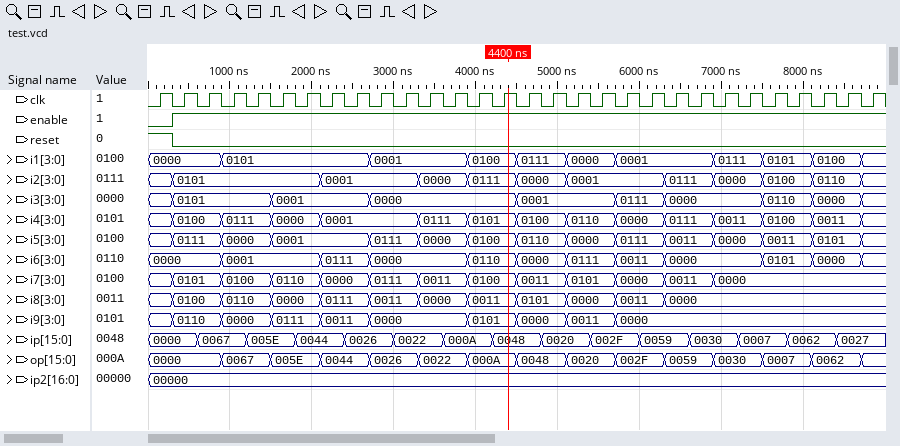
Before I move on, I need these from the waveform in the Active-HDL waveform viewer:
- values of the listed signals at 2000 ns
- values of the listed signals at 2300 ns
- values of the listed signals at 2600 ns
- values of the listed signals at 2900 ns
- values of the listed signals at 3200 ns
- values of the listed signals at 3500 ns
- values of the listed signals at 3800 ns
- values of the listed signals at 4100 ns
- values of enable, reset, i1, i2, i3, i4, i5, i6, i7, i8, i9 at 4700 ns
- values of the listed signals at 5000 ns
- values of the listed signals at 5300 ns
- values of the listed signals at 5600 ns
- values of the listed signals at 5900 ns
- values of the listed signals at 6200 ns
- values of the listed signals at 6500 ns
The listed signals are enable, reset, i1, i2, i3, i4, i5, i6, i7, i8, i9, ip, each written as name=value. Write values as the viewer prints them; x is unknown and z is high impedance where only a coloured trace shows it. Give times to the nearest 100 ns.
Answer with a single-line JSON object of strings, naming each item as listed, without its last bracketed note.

{"values of the listed signals at 2000 ns": "enable=1, reset=0, i1=0101, i2=0101, i3=0001, i4=0000, i5=0001, i6=0001, i7=0110, i8=0000, i9=0111, ip=0044", "values of the listed signals at 2300 ns": "enable=1, reset=0, i1=0101, i2=0001, i3=0001, i4=0001, i5=0001, i6=0111, i7=0000, i8=0111, i9=0011, ip=0044", "values of the listed signals at 2600 ns": "enable=1, reset=0, i1=0101, i2=0001, i3=0001, i4=0001, i5=0001, i6=0111, i7=0000, i8=0111, i9=0011, ip=0026", "values of the listed signals at 2900 ns": "enable=1, reset=0, i1=0001, i2=0001, i3=0000, i4=0001, i5=0111, i6=0000, i7=0111, i8=0011, i9=0000, ip=0026", "values of the listed signals at 3200 ns": "enable=1, reset=0, i1=0001, i2=0001, i3=0000, i4=0001, i5=0111, i6=0000, i7=0111, i8=0011, i9=0000, ip=0022", "values of the listed signals at 3500 ns": "enable=1, reset=0, i1=0001, i2=0000, i3=0000, i4=0111, i5=0000, i6=0000, i7=0011, i8=0000, i9=0000, ip=0022", "values of the listed signals at 3800 ns": "enable=1, reset=0, i1=0001, i2=0000, i3=0000, i4=0111, i5=0000, i6=0000, i7=0011, i8=0000, i9=0000, ip=000A", "values of the listed signals at 4100 ns": "enable=1, reset=0, i1=0100, i2=0111, i3=0000, i4=0101, i5=0100, i6=0110, i7=0100, i8=0011, i9=0101, ip=000A", "values of enable, reset, i1, i2, i3, i4, i5, i6, i7, i8, i9 at 4700 ns": "enable=1, reset=0, i1=0111, i2=0000, i3=0001, i4=0100, i5=0110, i6=0000, i7=0011, i8=0101, i9=0000", "values of the listed signals at 5000 ns": "enable=1, reset=0, i1=0111, i2=0000, i3=0001, i4=0100, i5=0110, i6=0000, i7=0011, i8=0101, i9=0000, ip=0020", "values of the listed signals at 5300 ns": "enable=1, reset=0, i1=0000, i2=0001, i3=0001, i4=0110, i5=0000, i6=0111, i7=0101, i8=0000, i9=0011, ip=0020", "values of the listed signals at 5600 ns": "enable=1, reset=0, i1=0000, i2=0001, i3=0001, i4=0110, i5=0000, i6=0111, i7=0101, i8=0000, i9=0011, ip=002F", "values of the listed signals at 5900 ns": "enable=1, reset=0, i1=0001, i2=0001, i3=0111, i4=0000, i5=0111, i6=0011, i7=0000, i8=0011, i9=0000, ip=002F", "values of the listed signals at 6200 ns": "enable=1, reset=0, i1=0001, i2=0001, i3=0111, i4=0000, i5=0111, i6=0011, i7=0000, i8=0011, i9=0000, ip=0059", "values of the listed signals at 6500 ns": "enable=1, reset=0, i1=0001, i2=0111, i3=0000, i4=0111, i5=0011, i6=0000, i7=0011, i8=0000, i9=0000, ip=0059"}
